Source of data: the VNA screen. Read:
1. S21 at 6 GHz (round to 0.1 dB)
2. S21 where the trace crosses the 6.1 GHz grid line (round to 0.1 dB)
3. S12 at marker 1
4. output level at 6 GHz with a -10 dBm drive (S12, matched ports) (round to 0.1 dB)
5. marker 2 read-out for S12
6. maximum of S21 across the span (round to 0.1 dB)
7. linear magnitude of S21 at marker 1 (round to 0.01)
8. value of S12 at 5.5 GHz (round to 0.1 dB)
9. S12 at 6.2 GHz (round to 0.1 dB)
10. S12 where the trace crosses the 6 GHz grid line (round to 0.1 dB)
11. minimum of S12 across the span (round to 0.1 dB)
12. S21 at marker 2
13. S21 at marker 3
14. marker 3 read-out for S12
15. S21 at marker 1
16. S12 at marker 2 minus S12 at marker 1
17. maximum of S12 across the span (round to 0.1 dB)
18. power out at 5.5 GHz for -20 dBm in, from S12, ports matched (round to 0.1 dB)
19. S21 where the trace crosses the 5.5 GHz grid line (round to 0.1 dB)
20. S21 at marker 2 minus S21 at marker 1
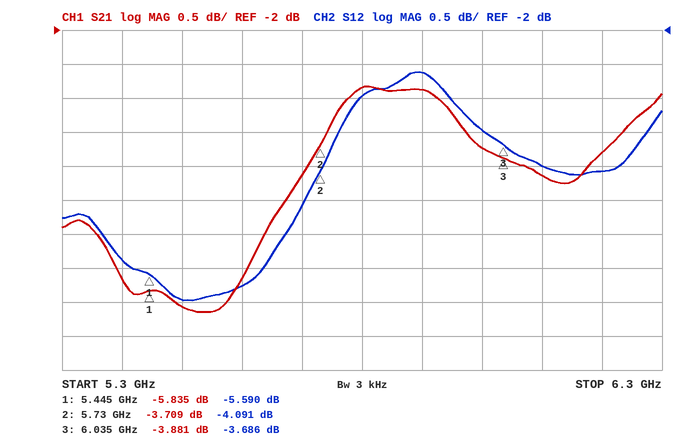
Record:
-3.7 dB
-4.1 dB
-5.590 dB
-13.5 dBm
-4.091 dB
-2.8 dB
0.51
-6.0 dB
-4.1 dB
-3.5 dB
-6.0 dB
-3.709 dB
-3.881 dB
-3.686 dB
-5.835 dB
1.499 dB
-2.6 dB
-26.0 dBm
-6.1 dB
2.126 dB
